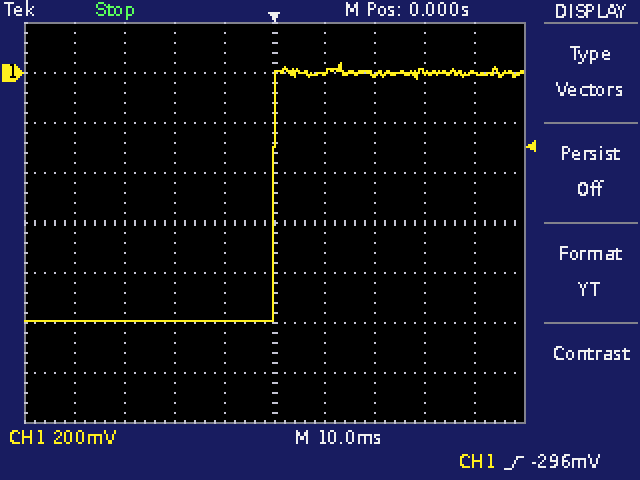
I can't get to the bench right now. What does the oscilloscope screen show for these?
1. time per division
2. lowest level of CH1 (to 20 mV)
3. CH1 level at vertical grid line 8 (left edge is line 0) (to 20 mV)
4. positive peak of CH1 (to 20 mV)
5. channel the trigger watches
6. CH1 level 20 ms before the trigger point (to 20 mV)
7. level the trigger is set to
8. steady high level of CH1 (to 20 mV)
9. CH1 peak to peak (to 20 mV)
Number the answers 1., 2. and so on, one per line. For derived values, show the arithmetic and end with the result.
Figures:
1. 10 ms
2. -1.00 V
3. 0 mV
4. 40 mV
5. CH1
6. -1.00 V
7. -296 mV
8. 0 mV
9. 40 mV − (-1.00 V) = 1.04 V
